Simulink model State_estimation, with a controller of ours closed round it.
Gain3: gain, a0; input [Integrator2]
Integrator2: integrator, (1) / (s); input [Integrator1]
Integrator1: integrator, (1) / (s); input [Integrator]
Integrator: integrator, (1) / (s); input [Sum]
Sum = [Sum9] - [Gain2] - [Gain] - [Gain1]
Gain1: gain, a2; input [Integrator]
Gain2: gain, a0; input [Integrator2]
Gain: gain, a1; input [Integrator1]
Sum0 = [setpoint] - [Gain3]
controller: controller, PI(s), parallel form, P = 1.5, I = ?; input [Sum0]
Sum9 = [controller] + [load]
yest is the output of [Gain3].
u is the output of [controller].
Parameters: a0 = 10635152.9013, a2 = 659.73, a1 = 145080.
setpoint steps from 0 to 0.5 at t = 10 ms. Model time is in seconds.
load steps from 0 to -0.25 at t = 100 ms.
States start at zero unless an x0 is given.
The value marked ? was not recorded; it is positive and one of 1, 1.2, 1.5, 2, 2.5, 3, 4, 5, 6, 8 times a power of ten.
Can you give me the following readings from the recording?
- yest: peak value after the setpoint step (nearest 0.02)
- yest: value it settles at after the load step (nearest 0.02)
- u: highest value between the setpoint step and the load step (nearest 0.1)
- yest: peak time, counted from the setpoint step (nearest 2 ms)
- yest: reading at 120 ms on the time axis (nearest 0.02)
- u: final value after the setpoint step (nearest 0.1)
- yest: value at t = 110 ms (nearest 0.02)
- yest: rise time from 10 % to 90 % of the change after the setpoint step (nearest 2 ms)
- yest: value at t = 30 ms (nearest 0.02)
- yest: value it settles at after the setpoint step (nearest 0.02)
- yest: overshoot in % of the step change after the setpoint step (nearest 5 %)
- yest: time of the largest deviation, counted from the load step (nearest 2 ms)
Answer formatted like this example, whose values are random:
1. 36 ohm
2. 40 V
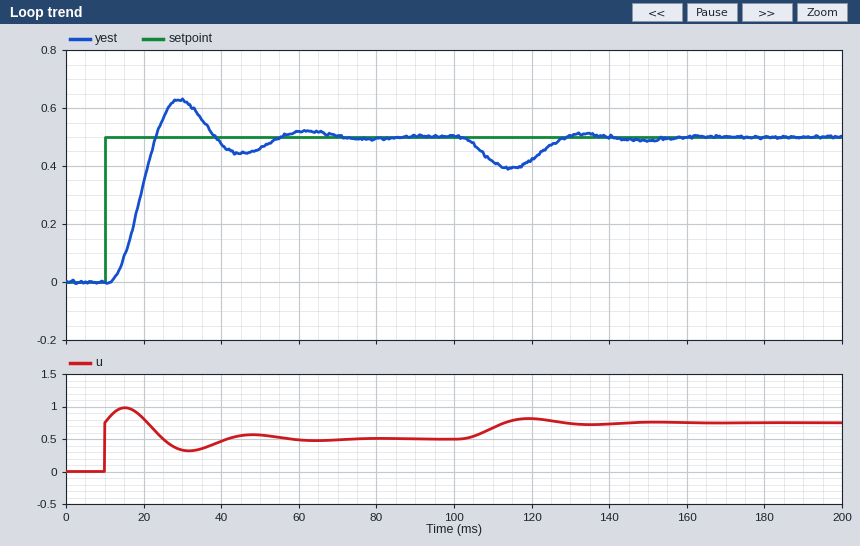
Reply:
1. 0.62
2. 0.50
3. 1.0
4. 20 ms
5. 0.42
6. 0.5
7. 0.42
8. 8 ms
9. 0.62
10. 0.50
11. 25 %
12. 14 ms
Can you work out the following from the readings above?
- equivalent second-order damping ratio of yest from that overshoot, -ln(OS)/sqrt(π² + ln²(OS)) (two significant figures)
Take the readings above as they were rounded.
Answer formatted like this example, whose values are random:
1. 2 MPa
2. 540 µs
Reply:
1. 0.40
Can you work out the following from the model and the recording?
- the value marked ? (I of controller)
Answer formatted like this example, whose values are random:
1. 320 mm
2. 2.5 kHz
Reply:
1. 150
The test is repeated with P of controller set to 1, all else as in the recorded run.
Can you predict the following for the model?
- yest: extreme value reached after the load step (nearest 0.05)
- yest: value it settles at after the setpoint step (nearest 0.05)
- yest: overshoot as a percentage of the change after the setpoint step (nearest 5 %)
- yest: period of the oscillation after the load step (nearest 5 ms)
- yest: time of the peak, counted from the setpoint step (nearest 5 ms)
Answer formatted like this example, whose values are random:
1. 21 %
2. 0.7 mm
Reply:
1. 0.40
2. 0.50
3. 30 %
4. 40 ms
5. 25 ms
